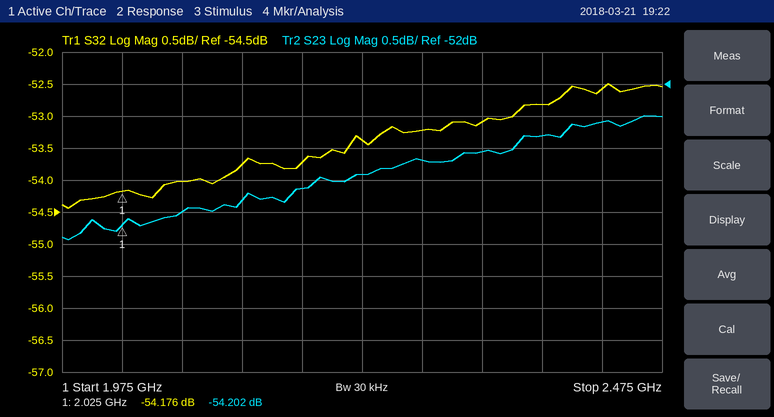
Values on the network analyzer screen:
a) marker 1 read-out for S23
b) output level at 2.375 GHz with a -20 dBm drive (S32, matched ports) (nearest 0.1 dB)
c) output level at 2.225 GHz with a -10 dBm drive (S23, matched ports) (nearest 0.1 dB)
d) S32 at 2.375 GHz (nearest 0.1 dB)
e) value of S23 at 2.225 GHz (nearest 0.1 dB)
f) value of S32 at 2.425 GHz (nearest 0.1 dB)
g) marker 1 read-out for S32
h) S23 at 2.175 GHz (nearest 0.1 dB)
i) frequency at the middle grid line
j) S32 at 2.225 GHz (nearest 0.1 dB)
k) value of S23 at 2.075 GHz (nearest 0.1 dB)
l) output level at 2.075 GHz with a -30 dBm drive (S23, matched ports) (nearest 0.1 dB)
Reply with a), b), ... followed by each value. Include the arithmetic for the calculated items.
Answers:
a) -54.202 dB
b) -20 dBm + (-52.8 dB) = -72.8 dBm
c) -10 dBm + (-53.4 dB) = -63.4 dBm
d) -52.8 dB
e) -53.4 dB
f) -52.6 dB
g) -54.176 dB
h) -53.6 dB
i) 2.225 GHz
j) -53.4 dB
k) -54.0 dB
l) -30 dBm + (-54.0 dB) = -84.0 dBm
